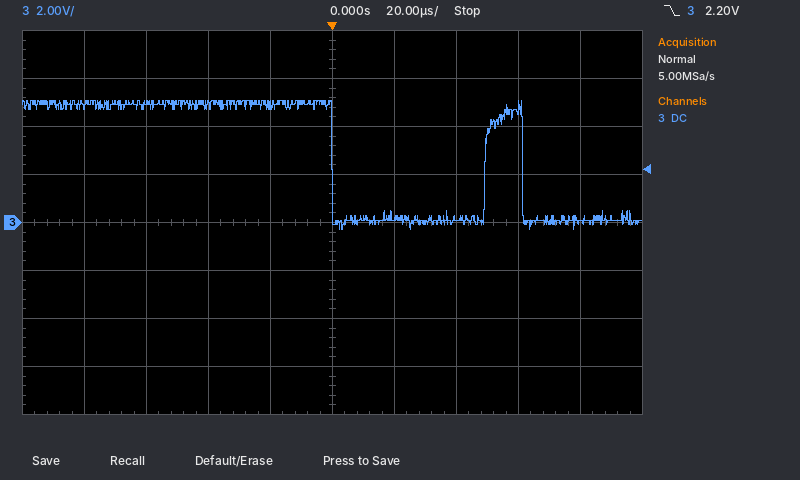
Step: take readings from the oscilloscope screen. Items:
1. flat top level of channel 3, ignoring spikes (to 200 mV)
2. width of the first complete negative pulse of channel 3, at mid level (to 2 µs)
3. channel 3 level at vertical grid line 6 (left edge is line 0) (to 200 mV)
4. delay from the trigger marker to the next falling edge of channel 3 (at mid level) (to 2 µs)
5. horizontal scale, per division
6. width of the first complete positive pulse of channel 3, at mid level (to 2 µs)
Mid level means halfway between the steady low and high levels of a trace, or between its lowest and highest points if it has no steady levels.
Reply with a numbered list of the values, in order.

1. 5.0 V
2. 50 µs
3. 200 mV
4. 62 µs
5. 20 µs
6. 12 µs
